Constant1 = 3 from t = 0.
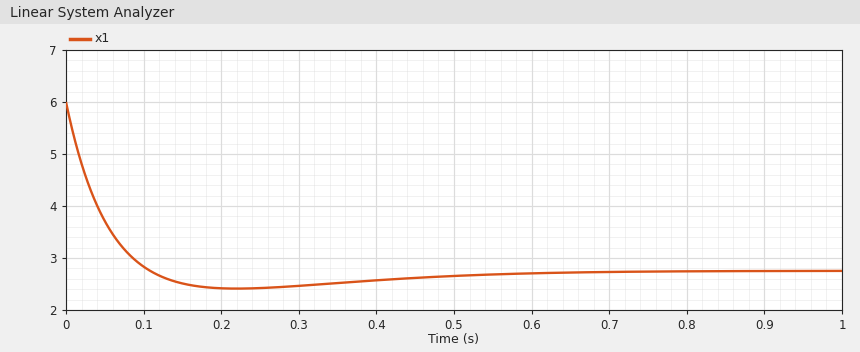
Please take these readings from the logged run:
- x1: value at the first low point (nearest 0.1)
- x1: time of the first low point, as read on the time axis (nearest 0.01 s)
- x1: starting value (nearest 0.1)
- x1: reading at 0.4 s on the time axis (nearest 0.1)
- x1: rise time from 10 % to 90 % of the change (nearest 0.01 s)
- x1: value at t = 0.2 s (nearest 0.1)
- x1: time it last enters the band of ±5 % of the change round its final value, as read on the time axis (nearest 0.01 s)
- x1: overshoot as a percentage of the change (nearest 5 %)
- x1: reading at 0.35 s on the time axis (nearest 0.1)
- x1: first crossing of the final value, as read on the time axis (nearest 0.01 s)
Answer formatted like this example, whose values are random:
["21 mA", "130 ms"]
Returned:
["2.4", "0.22 s", "6.0", "2.6", "0.08 s", "2.4", "0.42 s", "10 %", "2.5", "0.11 s"]
